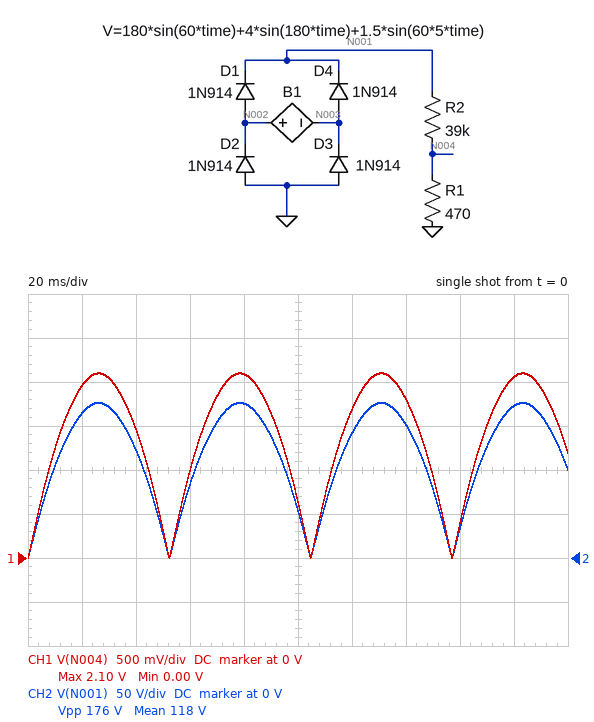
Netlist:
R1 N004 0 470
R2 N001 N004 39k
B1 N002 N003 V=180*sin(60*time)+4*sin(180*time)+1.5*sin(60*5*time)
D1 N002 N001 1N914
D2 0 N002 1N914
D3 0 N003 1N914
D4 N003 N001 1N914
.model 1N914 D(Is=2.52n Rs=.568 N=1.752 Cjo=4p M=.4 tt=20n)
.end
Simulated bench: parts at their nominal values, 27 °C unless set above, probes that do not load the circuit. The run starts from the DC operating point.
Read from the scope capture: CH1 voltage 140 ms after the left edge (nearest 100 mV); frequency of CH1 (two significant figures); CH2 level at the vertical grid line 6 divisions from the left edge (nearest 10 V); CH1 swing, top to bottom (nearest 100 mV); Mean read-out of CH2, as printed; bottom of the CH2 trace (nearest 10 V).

1.8 V
19 Hz
140 V
2.1 V
118 V
0 V
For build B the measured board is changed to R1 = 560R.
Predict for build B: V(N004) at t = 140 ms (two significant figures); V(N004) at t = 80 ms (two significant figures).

2.1 V
2.5 V
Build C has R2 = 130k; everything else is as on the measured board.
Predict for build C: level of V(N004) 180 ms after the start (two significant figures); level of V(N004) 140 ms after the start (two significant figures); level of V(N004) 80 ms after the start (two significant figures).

620 mV
550 mV
630 mV
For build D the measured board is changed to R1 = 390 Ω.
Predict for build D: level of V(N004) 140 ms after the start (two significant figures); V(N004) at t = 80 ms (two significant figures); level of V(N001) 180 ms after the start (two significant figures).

1.5 V
1.7 V
170 V
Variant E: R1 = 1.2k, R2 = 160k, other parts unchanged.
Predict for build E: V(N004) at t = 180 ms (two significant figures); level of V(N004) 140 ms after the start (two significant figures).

1.3 V
1.1 V
